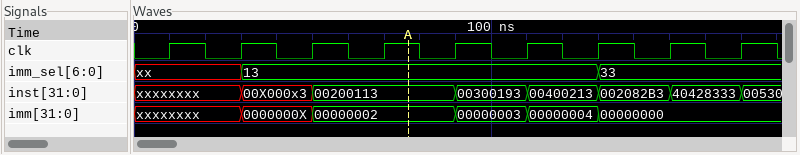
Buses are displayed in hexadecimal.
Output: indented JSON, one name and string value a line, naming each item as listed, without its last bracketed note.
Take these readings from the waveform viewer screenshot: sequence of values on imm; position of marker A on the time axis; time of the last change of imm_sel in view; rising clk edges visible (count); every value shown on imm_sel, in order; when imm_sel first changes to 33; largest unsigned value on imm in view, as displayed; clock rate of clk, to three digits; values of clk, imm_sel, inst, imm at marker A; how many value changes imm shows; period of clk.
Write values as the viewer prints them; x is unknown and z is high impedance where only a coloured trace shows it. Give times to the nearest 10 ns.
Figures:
{
  "sequence of values on imm": "xxxxxxxx, 0000000X, 00000002, 00000003, 00000004, 00000000",
  "position of marker A on the time axis": "80 ns",
  "time of the last change of imm_sel in view": "130 ns",
  "rising clk edges visible": "9",
  "every value shown on imm_sel, in order": "xx, 13, 33",
  "when imm_sel first changes to 33": "130 ns",
  "largest unsigned value on imm in view, as displayed": "00000004",
  "clock rate of clk, to three digits": "50.0 MHz",
  "values of clk, imm_sel, inst, imm at marker A": "clk=1, imm_sel=13, inst=00200113, imm=00000002",
  "how many value changes imm shows": "5",
  "period of clk": "20 ns"
}
